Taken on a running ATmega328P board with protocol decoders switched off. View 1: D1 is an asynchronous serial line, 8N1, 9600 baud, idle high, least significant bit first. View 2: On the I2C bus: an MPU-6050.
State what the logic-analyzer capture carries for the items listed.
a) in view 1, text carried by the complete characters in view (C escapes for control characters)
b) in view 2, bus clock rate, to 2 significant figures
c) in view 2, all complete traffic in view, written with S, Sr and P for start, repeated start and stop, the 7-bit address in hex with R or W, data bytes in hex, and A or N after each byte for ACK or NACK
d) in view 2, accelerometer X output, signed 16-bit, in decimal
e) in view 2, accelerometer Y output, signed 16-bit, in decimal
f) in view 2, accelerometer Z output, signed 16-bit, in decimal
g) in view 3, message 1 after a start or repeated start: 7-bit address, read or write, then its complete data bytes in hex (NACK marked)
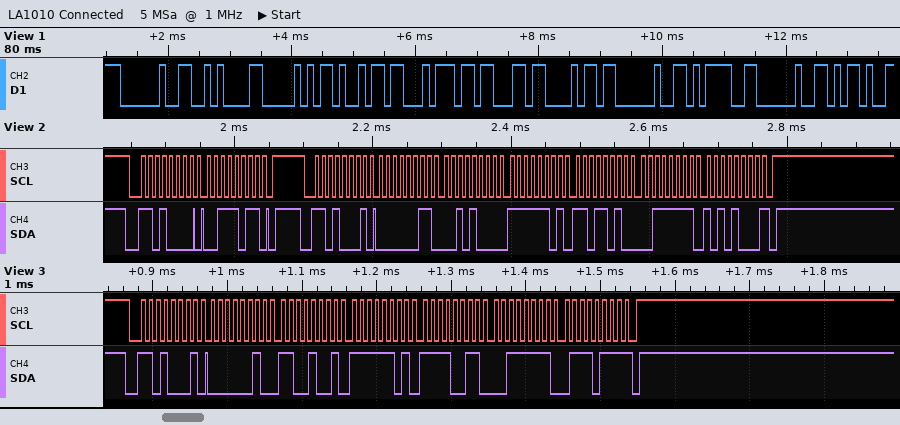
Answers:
" \nPitch = -"
100 kHz
S 68W A 3B A P S 68R A 03 A 28 A FD A DA A 3F A A8 N P
808
-550
16296
0x68 read: 02 C9 FD F3 3F 77 NACK
